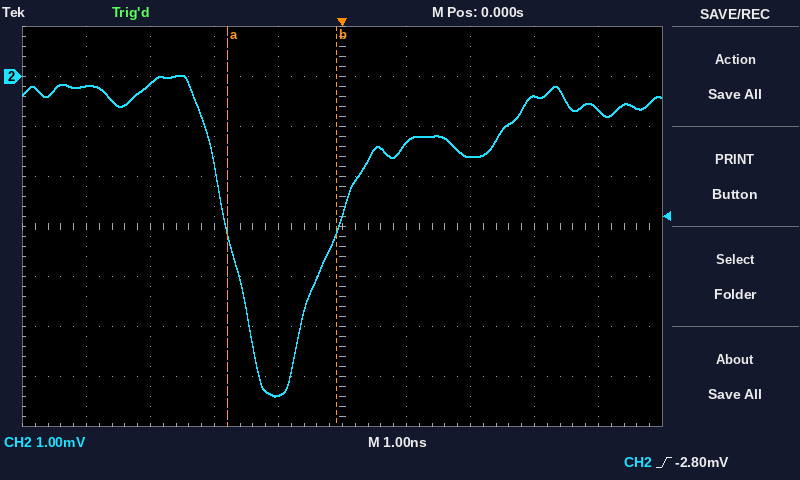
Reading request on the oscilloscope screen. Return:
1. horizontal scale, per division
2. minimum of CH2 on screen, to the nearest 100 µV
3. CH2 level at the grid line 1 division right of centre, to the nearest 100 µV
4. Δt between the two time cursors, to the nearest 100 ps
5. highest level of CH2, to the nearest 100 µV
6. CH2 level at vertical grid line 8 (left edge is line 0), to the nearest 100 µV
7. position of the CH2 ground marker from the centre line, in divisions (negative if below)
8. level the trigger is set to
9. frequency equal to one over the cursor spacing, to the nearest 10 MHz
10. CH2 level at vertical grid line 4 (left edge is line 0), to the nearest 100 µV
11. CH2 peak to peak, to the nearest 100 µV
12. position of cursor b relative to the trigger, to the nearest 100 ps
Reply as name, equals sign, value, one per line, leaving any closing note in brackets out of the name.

horizontal scale, per division = 1 ns
minimum of CH2 on screen, to the nearest 100 µV = -6.4 mV
CH2 level at the grid line 1 division right of centre, to the nearest 100 µV = -1.3 mV
Δt between the two time cursors, to the nearest 100 ps = 1.7 ns
highest level of CH2, to the nearest 100 µV = 0.0 mV
CH2 level at vertical grid line 8 (left edge is line 0), to the nearest 100 µV = -400 µV
position of the CH2 ground marker from the centre line, in divisions = +3.0 div
level the trigger is set to = -2.80 mV
frequency equal to one over the cursor spacing, to the nearest 10 MHz = 590 MHz
CH2 level at vertical grid line 4 (left edge is line 0), to the nearest 100 µV = -6.4 mV
CH2 peak to peak, to the nearest 100 µV = 6.4 mV
position of cursor b relative to the trigger, to the nearest 100 ps = -100 ps
